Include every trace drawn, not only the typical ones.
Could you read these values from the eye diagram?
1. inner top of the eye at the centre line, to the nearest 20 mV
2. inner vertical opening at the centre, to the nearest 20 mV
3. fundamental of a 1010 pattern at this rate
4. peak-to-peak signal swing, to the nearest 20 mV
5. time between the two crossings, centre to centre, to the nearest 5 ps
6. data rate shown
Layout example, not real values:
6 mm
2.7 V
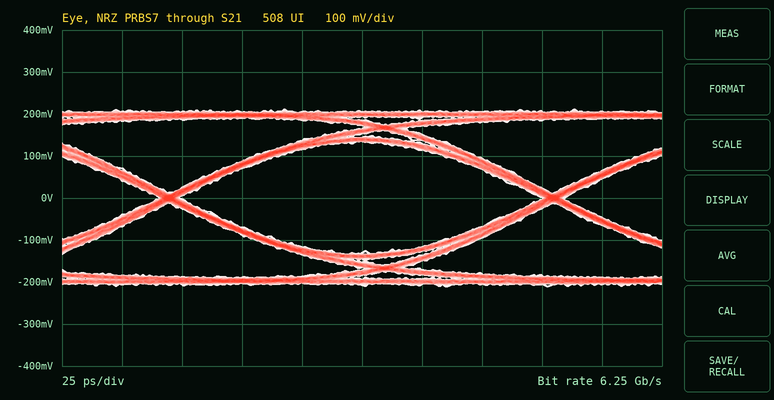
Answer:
140 mV
260 mV
3.125 GHz
420 mV
160 ps
6.25 Gb/s
